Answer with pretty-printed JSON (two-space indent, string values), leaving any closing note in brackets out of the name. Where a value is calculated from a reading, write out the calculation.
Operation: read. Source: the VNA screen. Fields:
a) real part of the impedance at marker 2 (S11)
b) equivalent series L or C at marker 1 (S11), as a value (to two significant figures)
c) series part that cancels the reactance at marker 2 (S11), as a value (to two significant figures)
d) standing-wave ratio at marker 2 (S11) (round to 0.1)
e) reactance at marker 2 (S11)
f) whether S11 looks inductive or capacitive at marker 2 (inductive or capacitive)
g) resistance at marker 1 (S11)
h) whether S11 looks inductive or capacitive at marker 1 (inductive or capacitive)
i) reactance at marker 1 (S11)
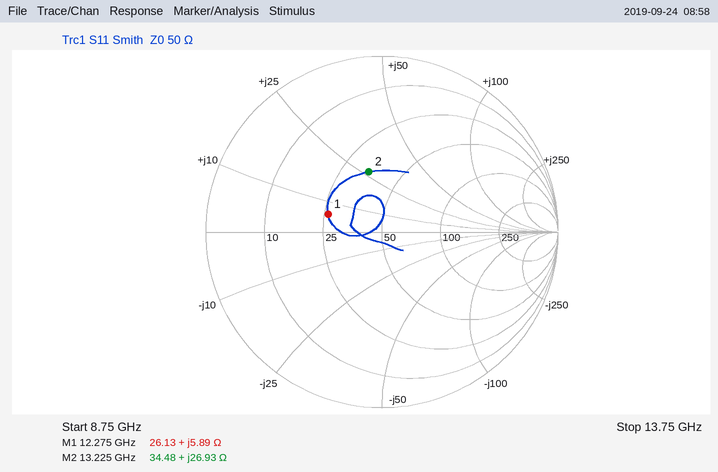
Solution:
{
  "real part of the impedance at marker 2": "34.48 Ω",
  "equivalent series L or C at marker 1 (S11), as a value": "L = 5.89 Ω/(2π × 12.275 GHz) ≈ 76 pH",
  "series part that cancels the reactance at marker 2 (S11), as a value": "C = 1/(2π × 13.225 GHz × 26.93 Ω) ≈ 447 fF, so 450 fF to two significant figures",
  "standing-wave ratio at marker 2 (S11)": "2.1",
  "reactance at marker 2": "+26.93 Ω",
  "whether S11 looks inductive or capacitive at marker 2": "inductive",
  "resistance at marker 1": "26.13 Ω",
  "whether S11 looks inductive or capacitive at marker 1": "inductive",
  "reactance at marker 1": "+5.89 Ω"
}
